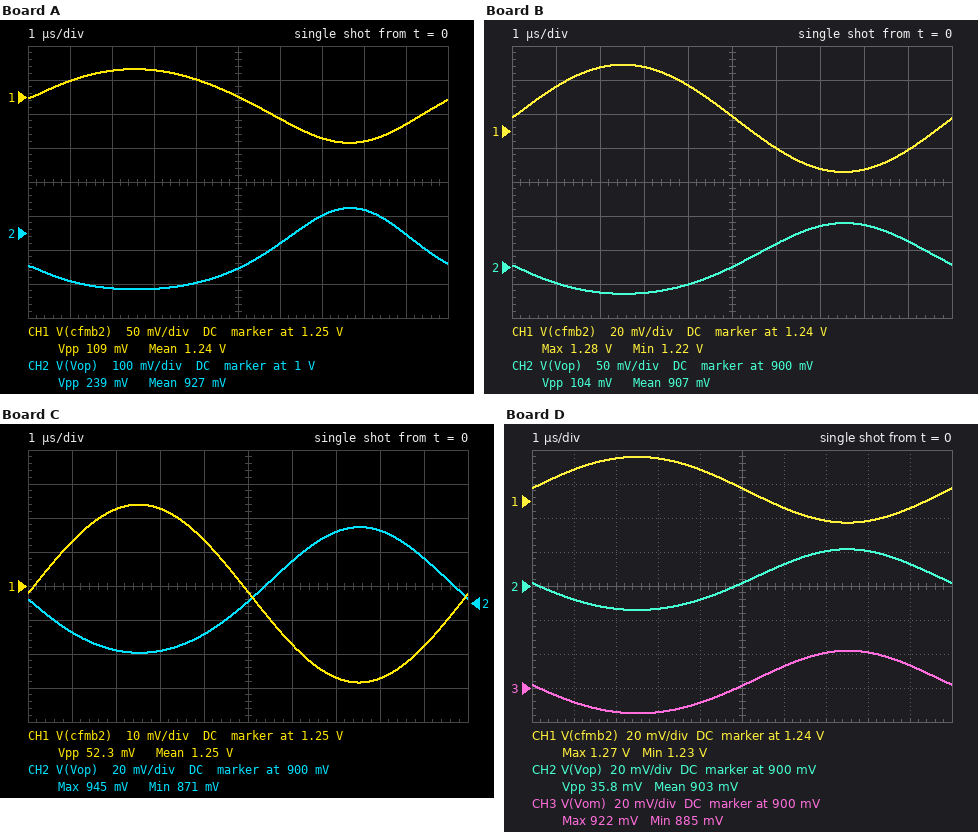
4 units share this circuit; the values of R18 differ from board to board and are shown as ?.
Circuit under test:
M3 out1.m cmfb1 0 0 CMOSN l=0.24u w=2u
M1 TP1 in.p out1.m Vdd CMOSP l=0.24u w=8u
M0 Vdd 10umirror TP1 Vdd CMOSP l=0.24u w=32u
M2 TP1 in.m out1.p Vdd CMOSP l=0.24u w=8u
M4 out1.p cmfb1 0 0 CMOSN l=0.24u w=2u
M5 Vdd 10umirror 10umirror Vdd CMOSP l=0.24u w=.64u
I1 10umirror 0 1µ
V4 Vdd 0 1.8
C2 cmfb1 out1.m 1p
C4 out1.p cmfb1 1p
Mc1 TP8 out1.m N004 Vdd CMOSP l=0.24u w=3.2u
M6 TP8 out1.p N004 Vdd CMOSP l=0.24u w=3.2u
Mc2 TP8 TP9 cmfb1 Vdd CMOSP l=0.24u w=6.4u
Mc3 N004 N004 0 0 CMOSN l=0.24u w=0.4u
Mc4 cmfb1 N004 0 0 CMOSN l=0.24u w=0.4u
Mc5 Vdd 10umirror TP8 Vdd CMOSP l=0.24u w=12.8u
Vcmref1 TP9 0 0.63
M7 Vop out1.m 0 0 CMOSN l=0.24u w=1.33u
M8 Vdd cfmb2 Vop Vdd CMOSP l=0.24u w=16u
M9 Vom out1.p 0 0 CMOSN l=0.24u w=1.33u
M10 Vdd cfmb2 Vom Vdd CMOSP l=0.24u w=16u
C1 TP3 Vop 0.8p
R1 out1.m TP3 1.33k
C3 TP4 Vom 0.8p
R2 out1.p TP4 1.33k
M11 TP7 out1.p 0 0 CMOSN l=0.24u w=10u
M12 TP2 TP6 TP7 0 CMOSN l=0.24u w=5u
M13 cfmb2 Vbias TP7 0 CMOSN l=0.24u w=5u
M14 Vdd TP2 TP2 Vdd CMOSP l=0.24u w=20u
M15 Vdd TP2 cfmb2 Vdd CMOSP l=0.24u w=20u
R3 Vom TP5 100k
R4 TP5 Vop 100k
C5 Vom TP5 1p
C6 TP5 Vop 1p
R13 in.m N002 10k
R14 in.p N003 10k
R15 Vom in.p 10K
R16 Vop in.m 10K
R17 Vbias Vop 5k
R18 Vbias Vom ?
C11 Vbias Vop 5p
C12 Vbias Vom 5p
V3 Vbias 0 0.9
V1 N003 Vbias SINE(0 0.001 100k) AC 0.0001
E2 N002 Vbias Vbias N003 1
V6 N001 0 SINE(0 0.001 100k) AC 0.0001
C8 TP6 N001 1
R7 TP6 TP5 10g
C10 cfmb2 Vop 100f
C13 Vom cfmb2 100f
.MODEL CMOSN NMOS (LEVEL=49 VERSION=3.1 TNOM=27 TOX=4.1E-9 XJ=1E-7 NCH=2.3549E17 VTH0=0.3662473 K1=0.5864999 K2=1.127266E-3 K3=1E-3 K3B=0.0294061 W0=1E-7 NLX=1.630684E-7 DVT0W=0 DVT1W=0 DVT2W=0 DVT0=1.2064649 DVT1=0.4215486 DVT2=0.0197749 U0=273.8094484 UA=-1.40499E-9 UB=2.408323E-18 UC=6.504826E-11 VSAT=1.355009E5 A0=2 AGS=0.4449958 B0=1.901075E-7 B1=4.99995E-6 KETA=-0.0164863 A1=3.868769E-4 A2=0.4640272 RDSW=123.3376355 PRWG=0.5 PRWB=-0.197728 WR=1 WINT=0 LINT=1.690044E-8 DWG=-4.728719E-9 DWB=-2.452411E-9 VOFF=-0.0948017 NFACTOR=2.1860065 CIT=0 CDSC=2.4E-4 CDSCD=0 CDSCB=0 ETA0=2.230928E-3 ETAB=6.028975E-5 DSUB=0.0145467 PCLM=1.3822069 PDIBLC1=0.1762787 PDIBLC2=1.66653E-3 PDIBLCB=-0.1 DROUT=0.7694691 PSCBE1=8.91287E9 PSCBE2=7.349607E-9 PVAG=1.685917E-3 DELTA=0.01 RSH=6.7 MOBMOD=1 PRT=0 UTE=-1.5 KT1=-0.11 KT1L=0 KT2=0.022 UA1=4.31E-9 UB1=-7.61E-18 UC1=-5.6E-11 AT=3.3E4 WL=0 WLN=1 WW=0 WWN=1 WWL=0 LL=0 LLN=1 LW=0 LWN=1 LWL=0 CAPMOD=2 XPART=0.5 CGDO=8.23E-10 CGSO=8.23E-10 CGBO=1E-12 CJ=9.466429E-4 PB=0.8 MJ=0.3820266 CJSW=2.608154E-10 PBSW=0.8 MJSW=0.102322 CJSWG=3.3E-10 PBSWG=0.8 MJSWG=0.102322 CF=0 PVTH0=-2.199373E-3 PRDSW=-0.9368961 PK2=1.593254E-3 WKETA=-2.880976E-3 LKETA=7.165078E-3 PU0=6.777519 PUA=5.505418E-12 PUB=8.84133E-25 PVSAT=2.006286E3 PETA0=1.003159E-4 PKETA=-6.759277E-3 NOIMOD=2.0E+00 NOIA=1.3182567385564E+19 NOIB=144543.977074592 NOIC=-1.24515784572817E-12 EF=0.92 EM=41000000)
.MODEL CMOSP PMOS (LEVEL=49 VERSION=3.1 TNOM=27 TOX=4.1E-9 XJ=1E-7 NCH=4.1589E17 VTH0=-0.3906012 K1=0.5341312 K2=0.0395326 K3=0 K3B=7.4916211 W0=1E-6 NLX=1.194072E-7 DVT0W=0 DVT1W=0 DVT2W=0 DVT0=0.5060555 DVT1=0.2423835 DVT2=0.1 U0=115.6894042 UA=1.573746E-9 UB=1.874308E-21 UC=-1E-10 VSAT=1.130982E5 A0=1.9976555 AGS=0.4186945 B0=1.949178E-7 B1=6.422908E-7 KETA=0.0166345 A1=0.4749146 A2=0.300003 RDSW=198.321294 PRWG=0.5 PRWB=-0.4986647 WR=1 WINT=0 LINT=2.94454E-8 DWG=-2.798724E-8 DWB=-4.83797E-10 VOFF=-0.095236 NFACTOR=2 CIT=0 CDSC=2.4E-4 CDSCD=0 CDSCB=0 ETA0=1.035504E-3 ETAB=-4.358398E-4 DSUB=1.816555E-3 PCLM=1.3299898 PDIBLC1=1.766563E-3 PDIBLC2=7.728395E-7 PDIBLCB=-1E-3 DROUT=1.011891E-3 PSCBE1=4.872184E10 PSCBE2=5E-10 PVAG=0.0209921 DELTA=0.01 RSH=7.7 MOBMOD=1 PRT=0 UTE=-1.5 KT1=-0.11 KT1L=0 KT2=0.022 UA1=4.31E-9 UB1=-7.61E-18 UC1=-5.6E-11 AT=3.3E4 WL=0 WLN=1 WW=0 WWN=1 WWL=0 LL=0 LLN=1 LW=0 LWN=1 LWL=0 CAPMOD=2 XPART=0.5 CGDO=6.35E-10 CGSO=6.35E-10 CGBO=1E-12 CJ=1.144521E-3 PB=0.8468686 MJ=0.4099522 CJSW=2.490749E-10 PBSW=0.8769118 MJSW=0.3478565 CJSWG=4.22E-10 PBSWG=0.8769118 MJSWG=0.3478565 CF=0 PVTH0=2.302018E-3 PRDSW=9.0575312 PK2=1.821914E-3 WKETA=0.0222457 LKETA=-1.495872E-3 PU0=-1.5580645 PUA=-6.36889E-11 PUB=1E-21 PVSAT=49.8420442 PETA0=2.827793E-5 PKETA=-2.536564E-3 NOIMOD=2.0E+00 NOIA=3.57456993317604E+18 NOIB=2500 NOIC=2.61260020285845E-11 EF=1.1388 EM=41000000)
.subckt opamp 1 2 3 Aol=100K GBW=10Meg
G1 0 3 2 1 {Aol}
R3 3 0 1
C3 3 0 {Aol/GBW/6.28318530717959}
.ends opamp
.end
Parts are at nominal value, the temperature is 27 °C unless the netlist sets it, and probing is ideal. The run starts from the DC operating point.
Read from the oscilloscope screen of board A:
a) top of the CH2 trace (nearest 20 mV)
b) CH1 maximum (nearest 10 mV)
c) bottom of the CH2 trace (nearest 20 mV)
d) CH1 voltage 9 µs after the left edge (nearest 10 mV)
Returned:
1.08 V
1.29 V
840 mV
1.21 V
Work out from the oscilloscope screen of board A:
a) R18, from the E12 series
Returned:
12 kΩ
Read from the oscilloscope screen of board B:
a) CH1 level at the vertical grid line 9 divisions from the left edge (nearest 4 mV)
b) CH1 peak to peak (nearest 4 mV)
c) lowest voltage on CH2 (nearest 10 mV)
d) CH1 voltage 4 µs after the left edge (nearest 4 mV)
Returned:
1.228 V
64 mV
860 mV
1.268 V
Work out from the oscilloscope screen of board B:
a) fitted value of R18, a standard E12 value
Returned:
5.6 kΩ
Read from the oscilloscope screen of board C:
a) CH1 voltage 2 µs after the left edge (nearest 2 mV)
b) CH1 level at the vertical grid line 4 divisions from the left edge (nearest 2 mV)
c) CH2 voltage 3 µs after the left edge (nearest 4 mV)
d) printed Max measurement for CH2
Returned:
1.272 V
1.264 V
872 mV
945 mV
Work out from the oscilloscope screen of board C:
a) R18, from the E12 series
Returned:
3.9 kΩ
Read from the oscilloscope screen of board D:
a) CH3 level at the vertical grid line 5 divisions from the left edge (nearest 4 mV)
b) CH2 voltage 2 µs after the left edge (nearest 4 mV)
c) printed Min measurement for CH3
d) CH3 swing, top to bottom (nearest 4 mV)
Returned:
900 mV
888 mV
885 mV
36 mV
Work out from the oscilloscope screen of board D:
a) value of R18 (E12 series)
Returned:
1.8 kΩ
